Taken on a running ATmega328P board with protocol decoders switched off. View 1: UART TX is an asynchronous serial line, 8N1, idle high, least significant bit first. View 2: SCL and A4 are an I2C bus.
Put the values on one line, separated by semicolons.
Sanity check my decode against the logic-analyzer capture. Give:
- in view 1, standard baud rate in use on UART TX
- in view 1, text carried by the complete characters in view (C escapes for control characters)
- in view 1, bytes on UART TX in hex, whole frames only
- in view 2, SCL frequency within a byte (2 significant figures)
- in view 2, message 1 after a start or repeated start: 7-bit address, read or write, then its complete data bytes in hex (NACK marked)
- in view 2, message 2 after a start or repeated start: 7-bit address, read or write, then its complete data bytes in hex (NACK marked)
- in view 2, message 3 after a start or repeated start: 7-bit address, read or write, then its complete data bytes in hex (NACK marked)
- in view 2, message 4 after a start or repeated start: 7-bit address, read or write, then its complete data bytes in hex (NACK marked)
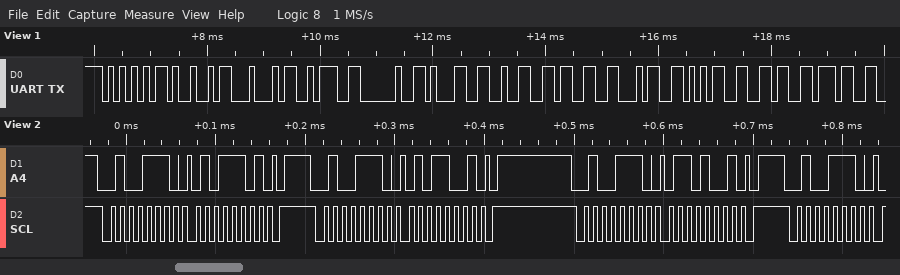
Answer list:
9600 baud; "UID: 1234567"; 0x55 0x49 0x44 0x3A 0x20 0x31 0x32 0x33 0x34 0x35 0x36 0x37; 100 kHz; 0x27 write: 5D; 0x27 write: 59; 0x27 write: 69; 0x27 write
